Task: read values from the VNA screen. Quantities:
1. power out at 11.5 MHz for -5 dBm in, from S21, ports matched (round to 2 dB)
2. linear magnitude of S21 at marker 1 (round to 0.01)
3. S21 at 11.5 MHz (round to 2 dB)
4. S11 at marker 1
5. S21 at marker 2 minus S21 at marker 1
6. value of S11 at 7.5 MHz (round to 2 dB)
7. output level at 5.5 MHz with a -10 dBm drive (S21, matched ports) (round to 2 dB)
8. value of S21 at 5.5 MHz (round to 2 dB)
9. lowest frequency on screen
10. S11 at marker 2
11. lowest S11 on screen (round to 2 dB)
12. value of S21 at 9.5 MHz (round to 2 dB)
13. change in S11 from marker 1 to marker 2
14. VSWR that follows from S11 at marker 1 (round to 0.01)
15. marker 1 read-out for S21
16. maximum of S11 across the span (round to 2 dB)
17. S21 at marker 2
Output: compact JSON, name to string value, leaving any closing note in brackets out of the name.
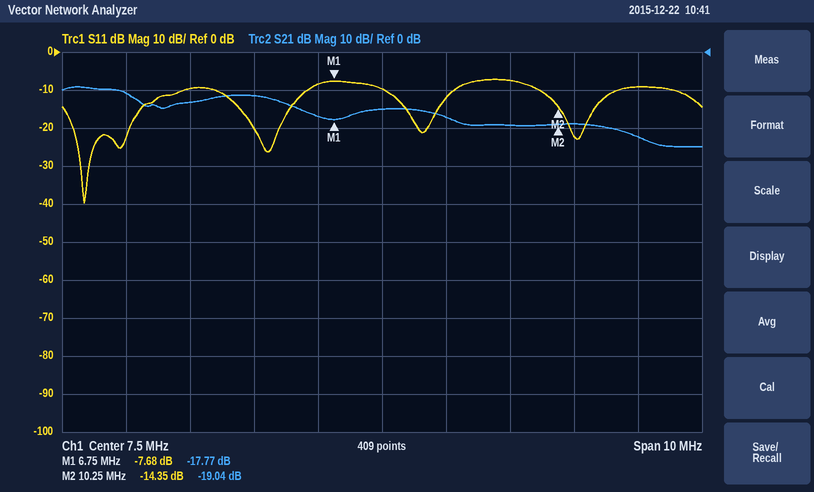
{"power out at 11.5 MHz for -5 dBm in, from S21, ports matched": "-28 dBm", "linear magnitude of S21 at marker 1": "0.13", "S21 at 11.5 MHz": "-22 dB", "S11 at marker 1": "-7.68 dB", "S21 at marker 2 minus S21 at marker 1": "-1.27 dB", "value of S11 at 7.5 MHz": "-10 dB", "output level at 5.5 MHz with a -10 dBm drive (S21, matched ports)": "-22 dBm", "value of S21 at 5.5 MHz": "-12 dB", "lowest frequency on screen": "2.5 MHz", "S11 at marker 2": "-14.35 dB", "lowest S11 on screen": "-40 dB", "value of S21 at 9.5 MHz": "-20 dB", "change in S11 from marker 1 to marker 2": "-6.67 dB", "VSWR that follows from S11 at marker 1": "2.41", "marker 1 read-out for S21": "-17.77 dB", "maximum of S11 across the span": "-8 dB", "S21 at marker 2": "-19.04 dB"}
